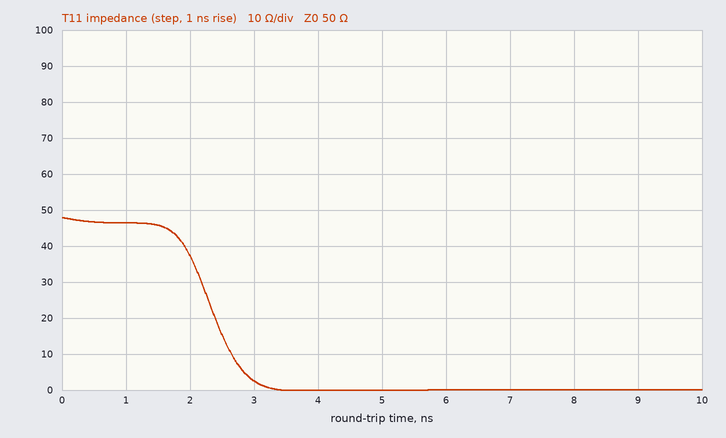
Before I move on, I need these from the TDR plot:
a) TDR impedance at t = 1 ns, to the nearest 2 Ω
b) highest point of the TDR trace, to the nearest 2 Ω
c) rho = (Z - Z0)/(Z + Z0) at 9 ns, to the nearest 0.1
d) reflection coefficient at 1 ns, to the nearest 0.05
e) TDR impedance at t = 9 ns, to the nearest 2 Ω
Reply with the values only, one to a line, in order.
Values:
46 Ω
48 Ω
-1.0
-0.05
0 Ω
